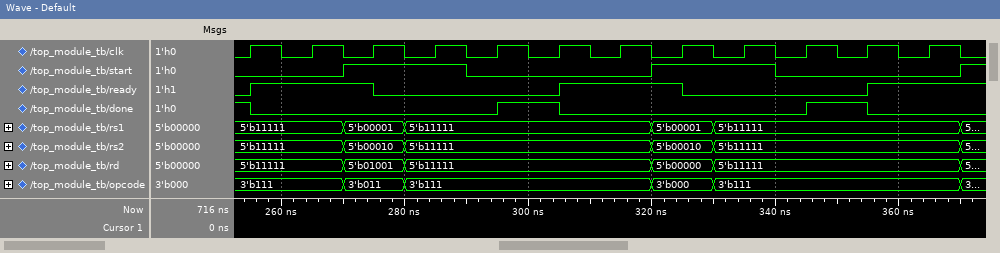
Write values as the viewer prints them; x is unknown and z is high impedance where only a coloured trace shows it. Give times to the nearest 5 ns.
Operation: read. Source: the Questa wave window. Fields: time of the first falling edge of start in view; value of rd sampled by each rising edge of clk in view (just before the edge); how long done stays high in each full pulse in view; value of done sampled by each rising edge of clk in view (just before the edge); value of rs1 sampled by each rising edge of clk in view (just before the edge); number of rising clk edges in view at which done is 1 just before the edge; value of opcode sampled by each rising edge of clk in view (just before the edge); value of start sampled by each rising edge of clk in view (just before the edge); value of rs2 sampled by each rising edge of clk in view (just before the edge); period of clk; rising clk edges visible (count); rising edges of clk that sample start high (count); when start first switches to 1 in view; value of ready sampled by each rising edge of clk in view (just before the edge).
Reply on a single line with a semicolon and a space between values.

290 ns; 5'b11111, 5'b11111, 5'b01001, 5'b11111, 5'b11111, 5'b11111, 5'b11111, 5'b00000, 5'b11111, 5'b11111, 5'b11111, 5'b11111; 10 ns, 10 ns; 1 0 0 0 0 1 0 0 0 0 1 0; 5'b11111, 5'b11111, 5'b00001, 5'b11111, 5'b11111, 5'b11111, 5'b11111, 5'b00001, 5'b11111, 5'b11111, 5'b11111, 5'b11111; 3; 3'b111, 3'b111, 3'b011, 3'b111, 3'b111, 3'b111, 3'b111, 3'b000, 3'b111, 3'b111, 3'b111, 3'b111; 0 0 1 1 0 0 0 1 1 0 0 0; 5'b11111, 5'b11111, 5'b00010, 5'b11111, 5'b11111, 5'b11111, 5'b11111, 5'b00010, 5'b11111, 5'b11111, 5'b11111, 5'b11111; 10 ns; 12; 4; 270 ns; 0 1 1 0 0 0 1 1 0 0 0 1
